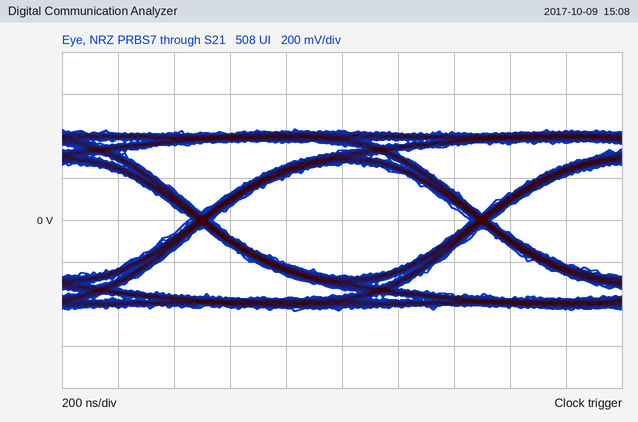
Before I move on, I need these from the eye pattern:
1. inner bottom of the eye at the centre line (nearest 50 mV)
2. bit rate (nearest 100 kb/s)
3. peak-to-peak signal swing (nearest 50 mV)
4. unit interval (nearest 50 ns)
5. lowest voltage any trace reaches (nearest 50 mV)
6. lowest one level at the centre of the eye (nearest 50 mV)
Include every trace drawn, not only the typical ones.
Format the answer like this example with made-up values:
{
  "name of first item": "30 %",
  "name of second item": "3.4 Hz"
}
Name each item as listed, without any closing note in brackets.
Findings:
{
  "inner bottom of the eye at the centre line": "-250 mV",
  "bit rate": "1.0 Mb/s",
  "peak-to-peak signal swing": "850 mV",
  "unit interval": "1.00 µs",
  "lowest voltage any trace reaches": "-450 mV",
  "lowest one level at the centre of the eye": "250 mV"
}
